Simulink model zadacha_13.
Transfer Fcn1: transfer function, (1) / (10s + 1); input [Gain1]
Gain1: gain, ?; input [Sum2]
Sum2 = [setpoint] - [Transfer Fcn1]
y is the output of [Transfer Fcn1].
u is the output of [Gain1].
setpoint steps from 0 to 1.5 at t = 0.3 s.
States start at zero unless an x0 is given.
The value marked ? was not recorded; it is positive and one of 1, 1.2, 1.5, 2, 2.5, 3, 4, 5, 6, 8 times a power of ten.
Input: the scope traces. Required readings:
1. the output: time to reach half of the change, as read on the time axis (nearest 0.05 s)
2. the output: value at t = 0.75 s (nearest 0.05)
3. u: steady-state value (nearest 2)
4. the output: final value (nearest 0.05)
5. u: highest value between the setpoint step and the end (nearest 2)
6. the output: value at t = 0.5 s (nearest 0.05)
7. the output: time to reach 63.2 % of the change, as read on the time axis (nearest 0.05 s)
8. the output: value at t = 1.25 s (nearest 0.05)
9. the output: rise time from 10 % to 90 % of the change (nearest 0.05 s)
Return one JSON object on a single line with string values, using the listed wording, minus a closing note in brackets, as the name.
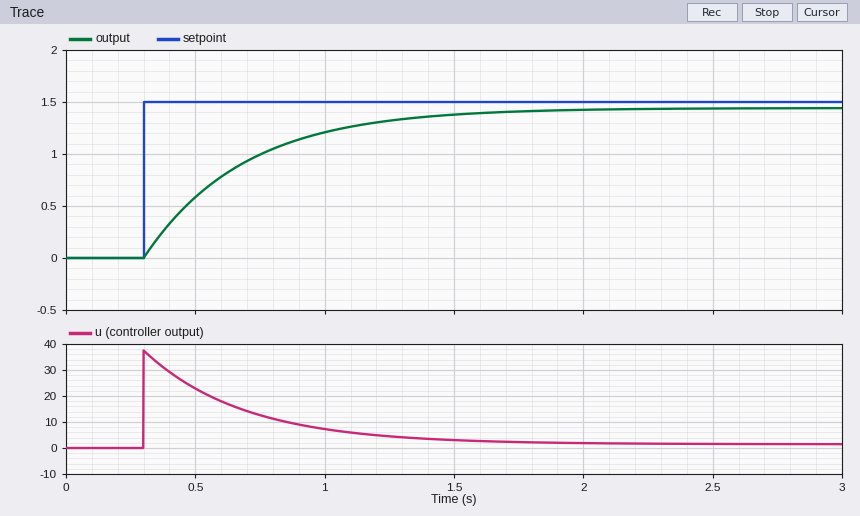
{"the output: time to reach half of the change, as read on the time axis": "0.55 s", "the output: value at t = 0.75 s": "1.00", "u: steady-state value": "2", "the output: final value": "1.45", "u: highest value between the setpoint step and the end": "38", "the output: value at t = 0.5 s": "0.60", "the output: time to reach 63.2 % of the change, as read on the time axis": "0.70 s", "the output: value at t = 1.25 s": "1.30", "the output: rise time from 10 % to 90 % of the change": "0.85 s"}
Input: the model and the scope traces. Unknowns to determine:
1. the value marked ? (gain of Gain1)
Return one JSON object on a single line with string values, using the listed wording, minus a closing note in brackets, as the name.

{"the value marked ?": "25"}
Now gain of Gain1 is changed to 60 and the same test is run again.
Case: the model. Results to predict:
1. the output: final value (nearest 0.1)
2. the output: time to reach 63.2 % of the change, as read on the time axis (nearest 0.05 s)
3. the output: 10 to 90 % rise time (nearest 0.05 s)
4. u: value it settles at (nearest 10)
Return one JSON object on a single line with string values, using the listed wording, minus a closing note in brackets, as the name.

{"the output: final value": "1.5", "the output: time to reach 63.2 % of the change, as read on the time axis": "0.45 s", "the output: 10 to 90 % rise time": "0.35 s", "u: value it settles at": "0"}
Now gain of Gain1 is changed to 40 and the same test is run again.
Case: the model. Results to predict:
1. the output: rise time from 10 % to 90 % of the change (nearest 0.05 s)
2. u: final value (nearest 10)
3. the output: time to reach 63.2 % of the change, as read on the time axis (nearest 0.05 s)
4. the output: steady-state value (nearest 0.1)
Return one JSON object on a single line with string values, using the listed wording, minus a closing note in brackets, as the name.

{"the output: rise time from 10 % to 90 % of the change": "0.55 s", "u: final value": "0", "the output: time to reach 63.2 % of the change, as read on the time axis": "0.55 s", "the output: steady-state value": "1.5"}
